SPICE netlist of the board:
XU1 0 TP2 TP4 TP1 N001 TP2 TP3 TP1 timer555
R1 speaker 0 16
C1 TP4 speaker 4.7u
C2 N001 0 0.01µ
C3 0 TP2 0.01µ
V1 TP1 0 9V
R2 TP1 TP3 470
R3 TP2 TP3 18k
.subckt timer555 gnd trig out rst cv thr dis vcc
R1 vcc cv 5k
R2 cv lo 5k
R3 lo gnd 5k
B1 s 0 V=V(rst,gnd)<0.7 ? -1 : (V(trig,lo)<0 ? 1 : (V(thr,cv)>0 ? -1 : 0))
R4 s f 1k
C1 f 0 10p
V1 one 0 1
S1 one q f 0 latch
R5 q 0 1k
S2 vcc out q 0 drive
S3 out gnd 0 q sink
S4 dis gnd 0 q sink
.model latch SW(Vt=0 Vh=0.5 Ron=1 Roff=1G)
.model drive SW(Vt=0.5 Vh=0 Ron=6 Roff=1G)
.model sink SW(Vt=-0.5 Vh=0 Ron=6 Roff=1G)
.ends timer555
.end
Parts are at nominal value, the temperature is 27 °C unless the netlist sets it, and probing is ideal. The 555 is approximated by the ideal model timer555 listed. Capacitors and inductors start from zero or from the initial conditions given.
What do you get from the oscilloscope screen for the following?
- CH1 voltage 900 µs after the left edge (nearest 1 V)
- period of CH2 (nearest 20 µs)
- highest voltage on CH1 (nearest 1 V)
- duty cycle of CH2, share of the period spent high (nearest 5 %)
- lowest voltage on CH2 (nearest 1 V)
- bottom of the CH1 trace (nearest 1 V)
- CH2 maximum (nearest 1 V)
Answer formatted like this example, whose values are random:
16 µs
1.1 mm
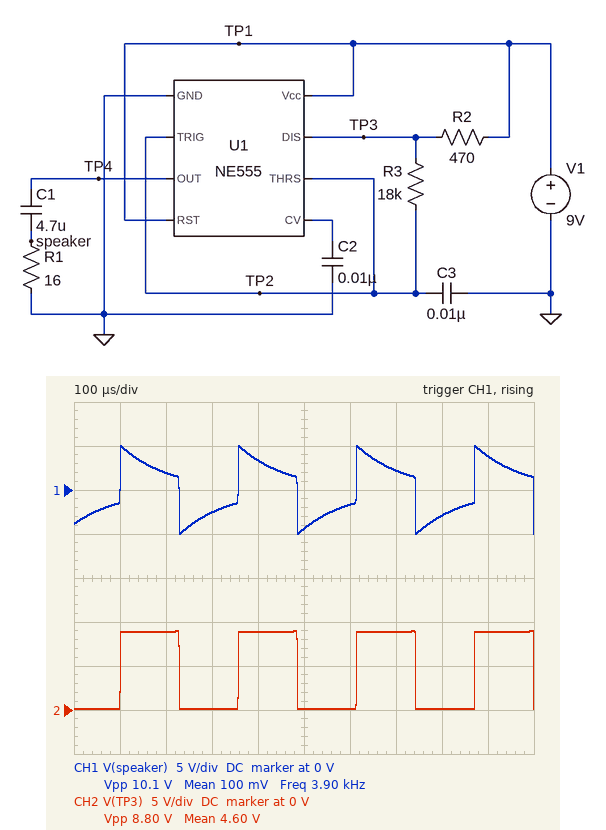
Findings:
4 V
260 µs
5 V
50 %
0 V
-5 V
9 V
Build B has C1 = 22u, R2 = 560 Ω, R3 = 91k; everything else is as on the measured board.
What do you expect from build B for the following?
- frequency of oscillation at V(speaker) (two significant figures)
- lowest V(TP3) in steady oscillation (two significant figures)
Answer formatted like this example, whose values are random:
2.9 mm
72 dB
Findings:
780 Hz
96 mV
